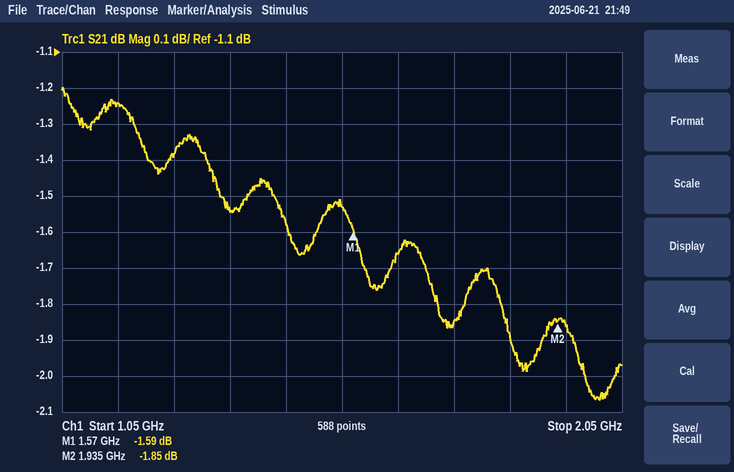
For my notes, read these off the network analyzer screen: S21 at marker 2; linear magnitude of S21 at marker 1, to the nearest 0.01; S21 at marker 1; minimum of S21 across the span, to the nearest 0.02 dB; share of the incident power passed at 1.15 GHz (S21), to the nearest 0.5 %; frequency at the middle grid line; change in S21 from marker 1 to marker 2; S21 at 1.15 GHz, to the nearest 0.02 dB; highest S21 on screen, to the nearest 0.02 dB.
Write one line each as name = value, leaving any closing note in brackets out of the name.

S21 at marker 2 = -1.85 dB
linear magnitude of S21 at marker 1, to the nearest 0.01 = 0.83
S21 at marker 1 = -1.59 dB
minimum of S21 across the span, to the nearest 0.02 dB = -2.06 dB
share of the incident power passed at 1.15 GHz (S21), to the nearest 0.5 % = 75.0 %
frequency at the middle grid line = 1.55 GHz
change in S21 from marker 1 to marker 2 = -0.26 dB
S21 at 1.15 GHz, to the nearest 0.02 dB = -1.24 dB
highest S21 on screen, to the nearest 0.02 dB = -1.20 dB
